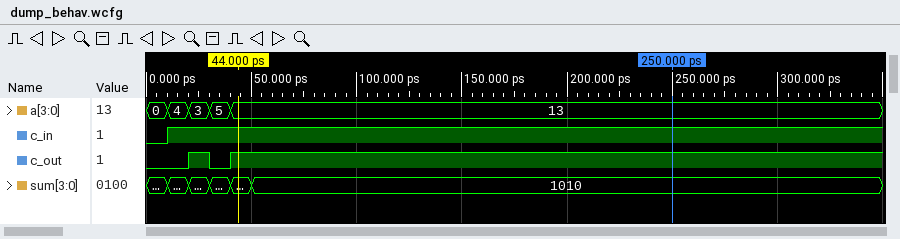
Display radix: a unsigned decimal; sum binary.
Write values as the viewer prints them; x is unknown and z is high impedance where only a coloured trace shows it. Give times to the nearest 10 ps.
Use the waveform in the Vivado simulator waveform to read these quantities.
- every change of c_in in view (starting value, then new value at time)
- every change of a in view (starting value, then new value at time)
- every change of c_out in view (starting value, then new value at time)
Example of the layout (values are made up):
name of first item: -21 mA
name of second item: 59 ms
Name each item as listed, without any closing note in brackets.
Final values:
every change of c_in in view: 0, 1 at 10 ps
every change of a in view: 0, 4 at 10 ps, 3 at 20 ps, 5 at 30 ps, 13 at 40 ps
every change of c_out in view: 0, 1 at 20 ps, 0 at 30 ps, 1 at 40 ps
